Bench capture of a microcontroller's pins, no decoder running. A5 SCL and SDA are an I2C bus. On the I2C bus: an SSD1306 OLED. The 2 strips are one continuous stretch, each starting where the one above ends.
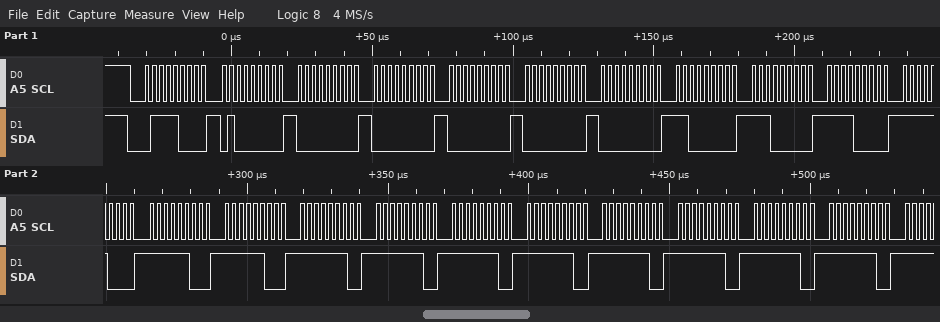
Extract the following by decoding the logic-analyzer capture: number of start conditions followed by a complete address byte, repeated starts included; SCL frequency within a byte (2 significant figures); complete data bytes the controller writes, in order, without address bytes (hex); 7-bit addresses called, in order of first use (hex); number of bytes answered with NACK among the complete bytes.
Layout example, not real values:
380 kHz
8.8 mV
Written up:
1
400 kHz
40 00 00 00 00 00 C0 E0 F0 F8 FC FC FE FE FE FE FE FE FE FE
0x3C
0
